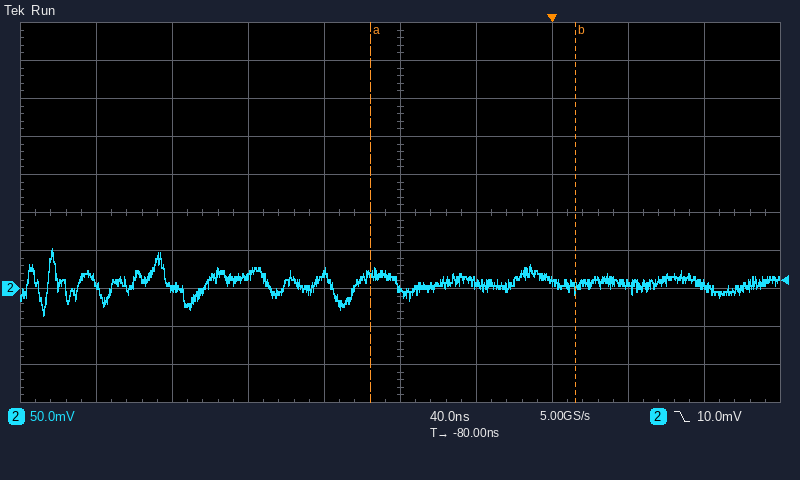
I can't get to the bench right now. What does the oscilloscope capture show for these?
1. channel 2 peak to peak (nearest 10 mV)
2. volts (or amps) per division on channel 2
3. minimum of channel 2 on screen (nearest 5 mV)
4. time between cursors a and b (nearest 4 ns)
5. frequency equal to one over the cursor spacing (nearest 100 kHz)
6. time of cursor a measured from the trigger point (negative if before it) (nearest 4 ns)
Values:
90 mV
50 mV
-35 mV
108 ns
9.3 MHz
-96 ns
